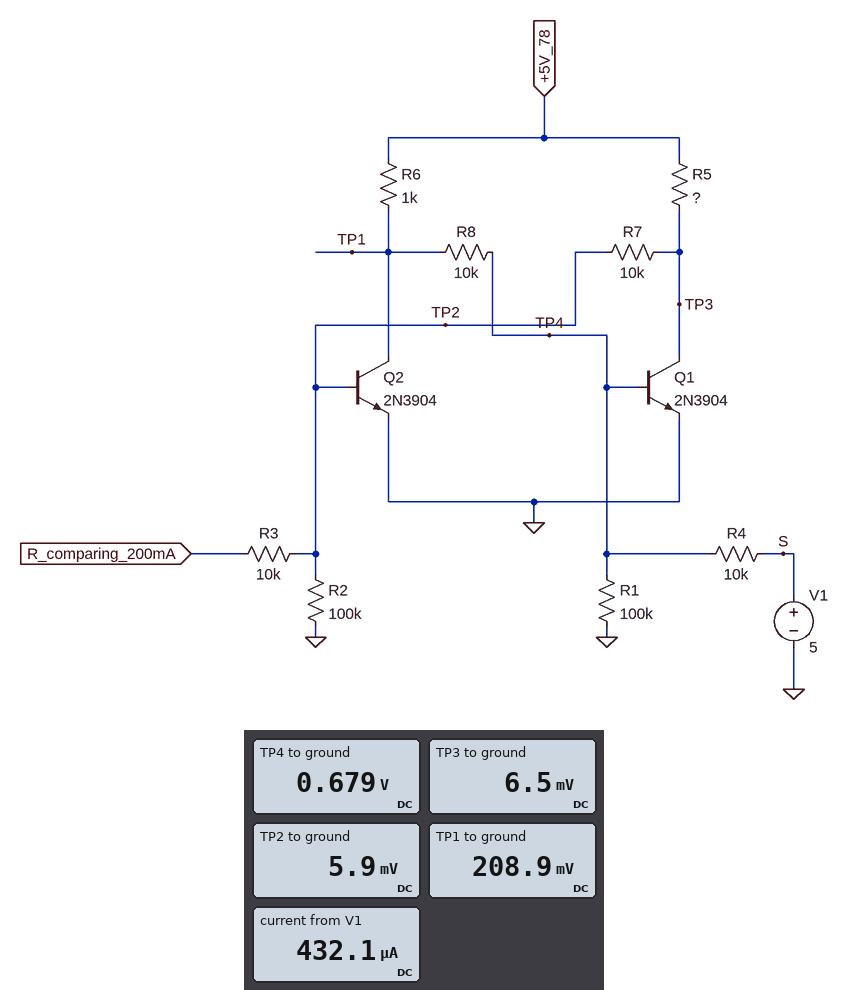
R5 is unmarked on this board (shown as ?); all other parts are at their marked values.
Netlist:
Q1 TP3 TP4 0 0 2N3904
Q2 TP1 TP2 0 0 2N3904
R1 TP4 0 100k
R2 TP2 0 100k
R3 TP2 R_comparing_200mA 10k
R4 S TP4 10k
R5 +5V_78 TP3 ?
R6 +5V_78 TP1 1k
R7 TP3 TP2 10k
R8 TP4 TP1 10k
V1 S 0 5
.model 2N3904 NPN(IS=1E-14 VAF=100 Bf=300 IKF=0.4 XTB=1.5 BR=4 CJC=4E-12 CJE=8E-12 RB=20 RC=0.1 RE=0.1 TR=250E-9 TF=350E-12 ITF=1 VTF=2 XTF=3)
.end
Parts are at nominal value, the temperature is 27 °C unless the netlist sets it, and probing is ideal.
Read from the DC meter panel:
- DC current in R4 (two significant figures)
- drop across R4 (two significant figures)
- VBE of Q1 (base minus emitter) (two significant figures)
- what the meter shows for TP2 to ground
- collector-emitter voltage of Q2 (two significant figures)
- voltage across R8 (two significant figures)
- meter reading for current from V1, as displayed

430 µA
4.3 V
680 mV
5.9 mV
210 mV
470 mV
432.1 µA
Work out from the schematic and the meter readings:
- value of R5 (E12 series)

3.3 kΩ
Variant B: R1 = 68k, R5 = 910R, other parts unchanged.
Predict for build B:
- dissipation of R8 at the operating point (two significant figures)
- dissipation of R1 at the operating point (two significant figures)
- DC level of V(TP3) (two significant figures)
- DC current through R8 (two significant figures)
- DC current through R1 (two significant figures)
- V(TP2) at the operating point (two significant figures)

32 µW
6.8 µW
6.7 mV
56 µA
10 µA
6.1 mV
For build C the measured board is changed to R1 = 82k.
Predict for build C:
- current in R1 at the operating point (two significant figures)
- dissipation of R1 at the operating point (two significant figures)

8.3 µA
5.6 µW
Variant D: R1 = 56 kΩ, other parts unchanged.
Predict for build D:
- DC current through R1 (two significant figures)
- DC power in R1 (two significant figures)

12 µA
8.2 µW
